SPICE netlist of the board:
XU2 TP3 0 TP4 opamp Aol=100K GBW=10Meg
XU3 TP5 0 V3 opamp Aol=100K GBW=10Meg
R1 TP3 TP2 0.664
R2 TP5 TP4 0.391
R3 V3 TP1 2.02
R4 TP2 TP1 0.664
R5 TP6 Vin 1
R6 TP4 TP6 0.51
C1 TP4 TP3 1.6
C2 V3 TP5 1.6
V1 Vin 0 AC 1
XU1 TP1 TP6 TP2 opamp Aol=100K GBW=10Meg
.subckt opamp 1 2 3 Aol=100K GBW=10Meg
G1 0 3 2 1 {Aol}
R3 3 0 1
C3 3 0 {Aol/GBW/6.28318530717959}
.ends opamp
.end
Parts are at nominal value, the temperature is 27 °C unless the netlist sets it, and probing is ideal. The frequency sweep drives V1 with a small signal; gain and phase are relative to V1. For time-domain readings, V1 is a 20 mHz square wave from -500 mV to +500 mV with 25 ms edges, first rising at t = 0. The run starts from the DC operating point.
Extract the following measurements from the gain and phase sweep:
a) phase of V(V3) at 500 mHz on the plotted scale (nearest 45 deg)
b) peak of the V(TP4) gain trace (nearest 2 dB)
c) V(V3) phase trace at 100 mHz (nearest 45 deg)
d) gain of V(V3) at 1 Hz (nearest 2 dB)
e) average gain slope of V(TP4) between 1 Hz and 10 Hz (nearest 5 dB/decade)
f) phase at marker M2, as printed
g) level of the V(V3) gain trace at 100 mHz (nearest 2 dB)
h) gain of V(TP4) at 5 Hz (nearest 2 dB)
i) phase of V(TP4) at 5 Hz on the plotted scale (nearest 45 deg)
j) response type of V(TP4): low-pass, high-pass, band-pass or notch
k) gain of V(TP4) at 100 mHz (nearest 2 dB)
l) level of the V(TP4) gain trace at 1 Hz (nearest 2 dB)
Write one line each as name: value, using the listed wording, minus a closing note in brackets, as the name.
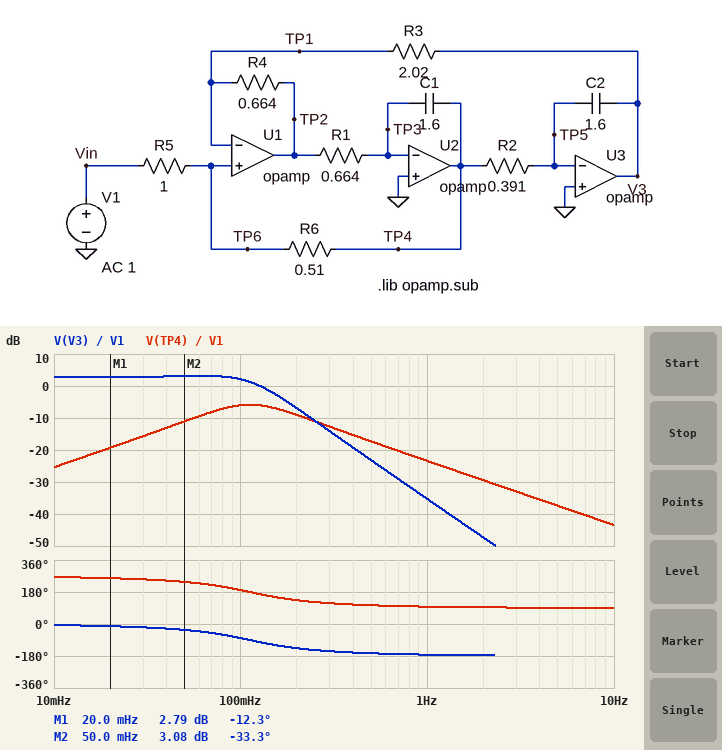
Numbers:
phase of V(V3) at 500 mHz on the plotted scale: -180 deg
peak of the V(TP4) gain trace: -6 dB
V(V3) phase trace at 100 mHz: -90 deg
gain of V(V3) at 1 Hz: -36 dB
average gain slope of V(TP4) between 1 Hz and 10 Hz: -20 dB/decade
phase at marker M2, as printed: -33.3 deg
level of the V(V3) gain trace at 100 mHz: 2 dB
gain of V(TP4) at 5 Hz: -38 dB
phase of V(TP4) at 5 Hz on the plotted scale: 90 deg
response type of V(TP4): low-pass, high-pass, band-pass or notch: band-pass
gain of V(TP4) at 100 mHz: -6 dB
level of the V(TP4) gain trace at 1 Hz: -24 dB
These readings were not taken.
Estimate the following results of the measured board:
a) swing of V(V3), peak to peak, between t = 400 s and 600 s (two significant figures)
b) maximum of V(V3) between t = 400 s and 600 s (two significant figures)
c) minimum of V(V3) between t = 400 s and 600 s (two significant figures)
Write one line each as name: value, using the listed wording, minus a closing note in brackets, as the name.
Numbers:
swing of V(V3), peak to peak, between t = 400 s and 600 s: 1.6 V
maximum of V(V3) between t = 400 s and 600 s: 820 mV
minimum of V(V3) between t = 400 s and 600 s: -820 mV
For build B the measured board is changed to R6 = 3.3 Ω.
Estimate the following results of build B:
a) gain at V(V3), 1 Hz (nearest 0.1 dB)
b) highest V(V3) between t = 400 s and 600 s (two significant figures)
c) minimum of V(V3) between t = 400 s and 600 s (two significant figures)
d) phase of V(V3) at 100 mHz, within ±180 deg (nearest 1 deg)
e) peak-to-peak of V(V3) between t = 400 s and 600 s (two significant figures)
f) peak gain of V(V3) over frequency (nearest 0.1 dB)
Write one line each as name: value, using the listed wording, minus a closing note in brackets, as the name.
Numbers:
gain at V(V3), 1 Hz: -28.1 dB
highest V(V3) between t = 400 s and 600 s: 3.2 V
minimum of V(V3) between t = 400 s and 600 s: -3.2 V
phase of V(V3) at 100 mHz, within ±180 deg: -61 deg
peak-to-peak of V(V3) between t = 400 s and 600 s: 6.3 V
peak gain of V(V3) over frequency: 17.7 dB
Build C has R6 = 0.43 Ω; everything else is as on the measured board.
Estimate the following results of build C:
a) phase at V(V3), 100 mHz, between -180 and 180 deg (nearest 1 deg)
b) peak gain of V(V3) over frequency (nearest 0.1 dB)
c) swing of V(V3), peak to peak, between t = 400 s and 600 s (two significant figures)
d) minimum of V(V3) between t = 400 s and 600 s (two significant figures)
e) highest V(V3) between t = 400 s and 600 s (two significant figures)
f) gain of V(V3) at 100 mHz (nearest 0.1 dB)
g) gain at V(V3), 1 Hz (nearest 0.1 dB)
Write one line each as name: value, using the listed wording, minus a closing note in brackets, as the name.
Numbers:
phase at V(V3), 100 mHz, between -180 and 180 deg: -80 deg
peak gain of V(V3) over frequency: 1.9 dB
swing of V(V3), peak to peak, between t = 400 s and 600 s: 1.4 V
minimum of V(V3) between t = 400 s and 600 s: -710 mV
highest V(V3) between t = 400 s and 600 s: 710 mV
gain of V(V3) at 100 mHz: 0.6 dB
gain at V(V3), 1 Hz: -36.3 dB
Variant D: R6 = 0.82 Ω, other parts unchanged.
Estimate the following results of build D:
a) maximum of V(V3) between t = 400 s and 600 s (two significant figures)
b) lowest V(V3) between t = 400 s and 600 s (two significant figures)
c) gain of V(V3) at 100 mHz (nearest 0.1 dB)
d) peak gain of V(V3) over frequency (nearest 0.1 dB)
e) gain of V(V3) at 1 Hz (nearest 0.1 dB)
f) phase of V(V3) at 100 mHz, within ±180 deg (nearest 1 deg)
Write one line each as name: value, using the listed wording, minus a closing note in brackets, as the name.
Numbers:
maximum of V(V3) between t = 400 s and 600 s: 1.2 V
lowest V(V3) between t = 400 s and 600 s: -1.2 V
gain of V(V3) at 100 mHz: 6.2 dB
peak gain of V(V3) over frequency: 6.6 dB
gain of V(V3) at 1 Hz: -32.8 dB
phase of V(V3) at 100 mHz, within ±180 deg: -77 deg
